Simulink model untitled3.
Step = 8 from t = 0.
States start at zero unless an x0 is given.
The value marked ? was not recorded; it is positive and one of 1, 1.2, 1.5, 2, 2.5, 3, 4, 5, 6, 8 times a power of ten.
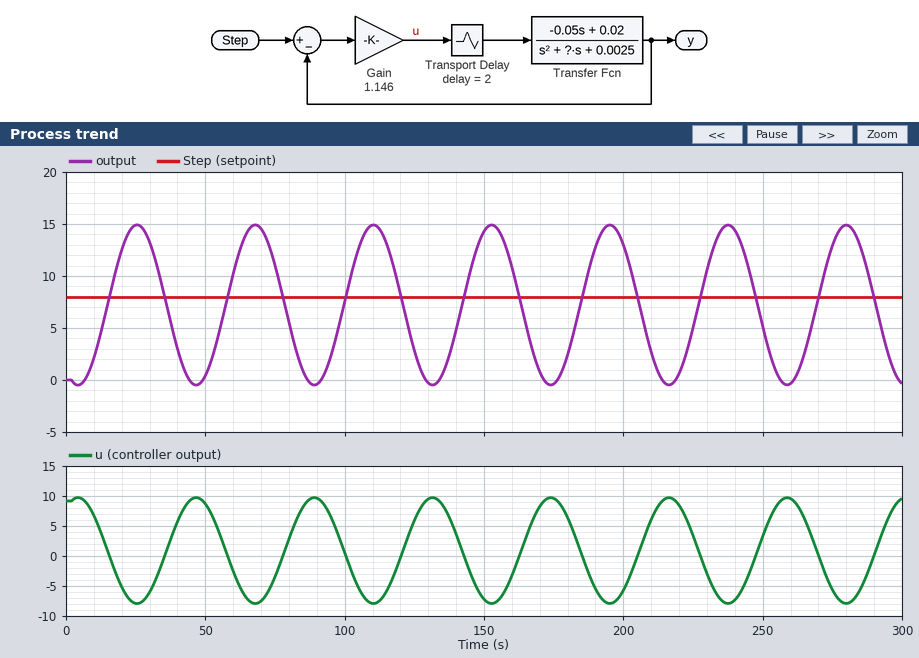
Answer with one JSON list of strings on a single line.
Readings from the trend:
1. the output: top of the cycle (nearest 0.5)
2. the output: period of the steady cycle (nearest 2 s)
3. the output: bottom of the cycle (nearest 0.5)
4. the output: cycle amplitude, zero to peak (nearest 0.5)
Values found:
["15.0", "42 s", "-0.5", "7.5"]
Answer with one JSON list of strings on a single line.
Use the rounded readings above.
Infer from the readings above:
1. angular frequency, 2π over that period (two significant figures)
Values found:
["0.15 rad/s"]
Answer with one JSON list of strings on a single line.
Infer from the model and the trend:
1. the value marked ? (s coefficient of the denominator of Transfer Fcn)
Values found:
["0.1"]
